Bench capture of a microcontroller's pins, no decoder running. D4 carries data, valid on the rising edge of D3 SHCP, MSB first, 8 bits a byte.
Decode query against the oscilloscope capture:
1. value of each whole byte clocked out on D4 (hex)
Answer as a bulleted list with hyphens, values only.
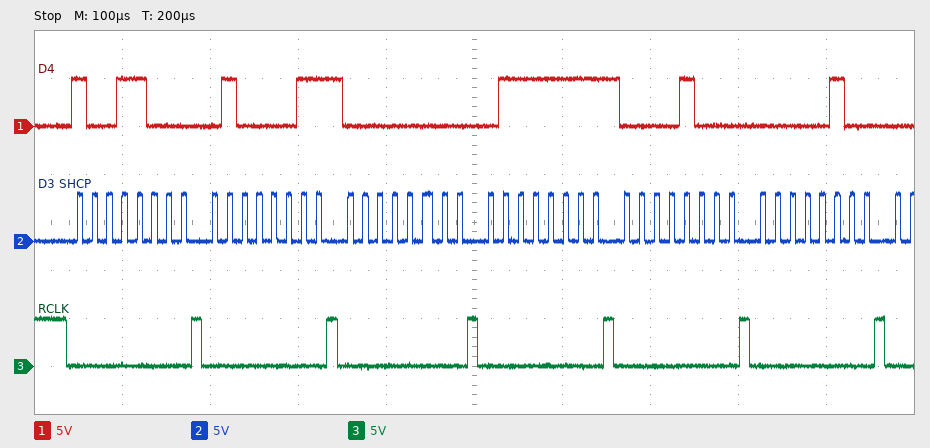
- 98 43 00 7F 08 04
